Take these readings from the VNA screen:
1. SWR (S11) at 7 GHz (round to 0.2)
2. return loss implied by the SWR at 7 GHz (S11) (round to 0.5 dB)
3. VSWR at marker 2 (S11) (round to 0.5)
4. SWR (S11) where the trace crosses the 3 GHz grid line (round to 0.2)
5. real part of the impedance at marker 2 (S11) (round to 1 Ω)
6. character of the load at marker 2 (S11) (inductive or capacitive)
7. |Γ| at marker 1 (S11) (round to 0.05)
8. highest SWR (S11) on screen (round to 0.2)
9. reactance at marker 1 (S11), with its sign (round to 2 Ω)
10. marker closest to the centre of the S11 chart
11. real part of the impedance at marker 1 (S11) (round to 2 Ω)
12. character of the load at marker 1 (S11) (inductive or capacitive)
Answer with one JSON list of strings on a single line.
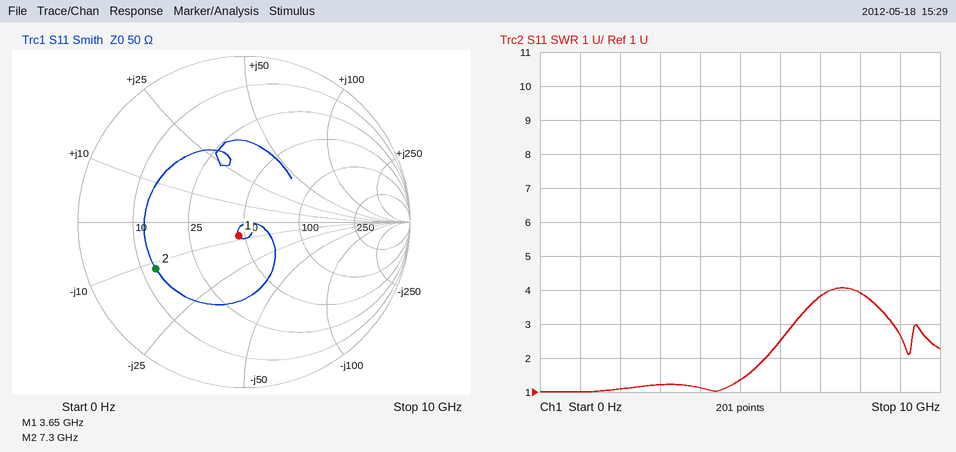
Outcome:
["3.8", "4.5 dB", "4.0", "1.2", "13 Ω", "capacitive", "0.10", "4.0", "-8 Ω", "marker 1", "46 Ω", "capacitive"]
